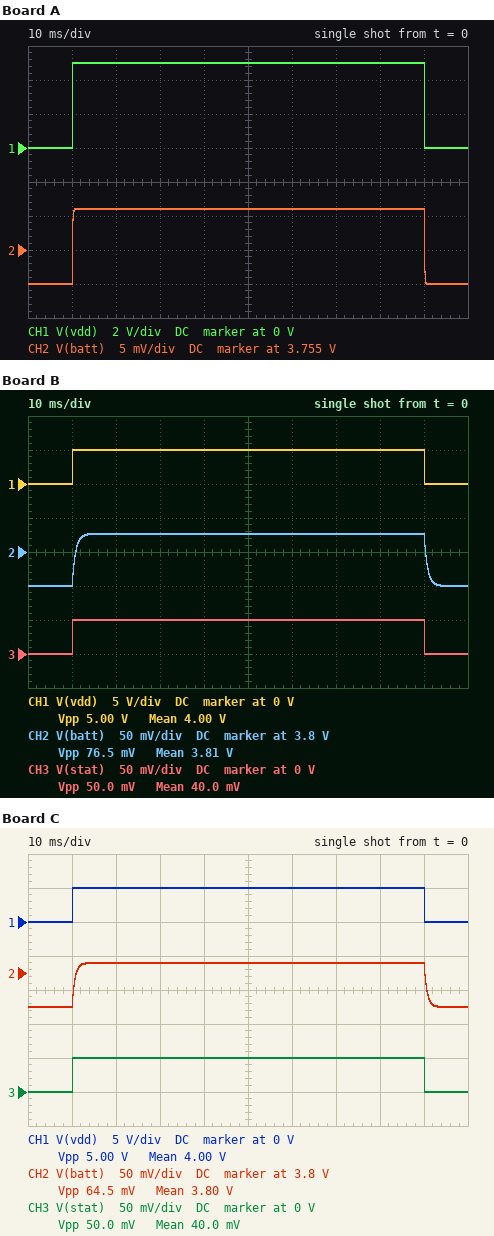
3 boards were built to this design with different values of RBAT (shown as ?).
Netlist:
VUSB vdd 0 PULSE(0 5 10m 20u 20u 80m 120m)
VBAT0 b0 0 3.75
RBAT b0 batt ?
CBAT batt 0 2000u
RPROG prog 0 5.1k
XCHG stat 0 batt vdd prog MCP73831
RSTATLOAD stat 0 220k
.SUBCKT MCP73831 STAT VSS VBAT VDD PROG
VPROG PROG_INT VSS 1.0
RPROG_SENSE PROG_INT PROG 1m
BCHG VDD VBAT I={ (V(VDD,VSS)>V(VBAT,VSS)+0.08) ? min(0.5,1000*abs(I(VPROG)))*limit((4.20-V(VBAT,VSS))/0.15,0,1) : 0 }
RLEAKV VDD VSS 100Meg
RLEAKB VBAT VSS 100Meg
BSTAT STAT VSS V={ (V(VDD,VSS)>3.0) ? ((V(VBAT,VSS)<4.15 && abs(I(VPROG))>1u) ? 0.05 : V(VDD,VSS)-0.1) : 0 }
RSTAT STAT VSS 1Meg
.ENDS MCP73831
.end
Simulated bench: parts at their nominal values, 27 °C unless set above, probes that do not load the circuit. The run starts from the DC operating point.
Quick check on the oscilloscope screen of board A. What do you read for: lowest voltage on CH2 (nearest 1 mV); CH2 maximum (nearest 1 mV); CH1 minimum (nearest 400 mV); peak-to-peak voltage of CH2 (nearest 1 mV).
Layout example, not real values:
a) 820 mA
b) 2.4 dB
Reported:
a) 3.750 V
b) 3.761 V
c) 0 V
d) 11 mV
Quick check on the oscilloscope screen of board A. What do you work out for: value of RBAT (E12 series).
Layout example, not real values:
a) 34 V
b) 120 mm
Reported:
a) 0.056 Ω
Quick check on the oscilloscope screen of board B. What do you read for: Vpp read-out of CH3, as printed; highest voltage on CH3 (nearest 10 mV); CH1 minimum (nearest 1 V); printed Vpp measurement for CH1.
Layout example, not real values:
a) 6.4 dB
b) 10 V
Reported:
a) 50.0 mV
b) 50 mV
c) 0 V
d) 5.00 V
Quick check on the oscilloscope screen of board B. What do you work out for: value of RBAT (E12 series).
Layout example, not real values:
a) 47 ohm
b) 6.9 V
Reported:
a) 0.39 Ω
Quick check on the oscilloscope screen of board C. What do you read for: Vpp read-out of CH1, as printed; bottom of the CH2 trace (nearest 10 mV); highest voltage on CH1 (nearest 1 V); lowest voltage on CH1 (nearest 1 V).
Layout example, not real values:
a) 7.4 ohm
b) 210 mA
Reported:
a) 5.00 V
b) 3.75 V
c) 5 V
d) 0 V
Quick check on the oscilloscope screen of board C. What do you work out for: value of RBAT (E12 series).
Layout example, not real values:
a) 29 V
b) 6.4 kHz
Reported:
a) 0.33 Ω
